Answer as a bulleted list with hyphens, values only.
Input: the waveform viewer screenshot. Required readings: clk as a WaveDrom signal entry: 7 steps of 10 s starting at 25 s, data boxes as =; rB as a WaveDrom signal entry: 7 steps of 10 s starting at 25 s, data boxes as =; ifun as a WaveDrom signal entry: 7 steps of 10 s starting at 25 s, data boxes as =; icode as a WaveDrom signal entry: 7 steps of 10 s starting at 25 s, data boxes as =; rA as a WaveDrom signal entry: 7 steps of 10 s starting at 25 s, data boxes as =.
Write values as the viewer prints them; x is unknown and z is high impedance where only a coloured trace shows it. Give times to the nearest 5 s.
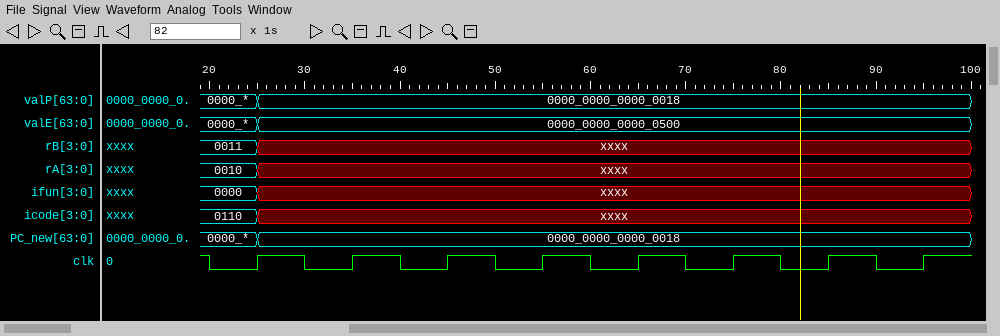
- {name: 'clk', wave: 'p......'}
- {name: 'rB', wave: 'x......'}
- {name: 'ifun', wave: 'x......'}
- {name: 'icode', wave: 'x......'}
- {name: 'rA', wave: 'x......'}
